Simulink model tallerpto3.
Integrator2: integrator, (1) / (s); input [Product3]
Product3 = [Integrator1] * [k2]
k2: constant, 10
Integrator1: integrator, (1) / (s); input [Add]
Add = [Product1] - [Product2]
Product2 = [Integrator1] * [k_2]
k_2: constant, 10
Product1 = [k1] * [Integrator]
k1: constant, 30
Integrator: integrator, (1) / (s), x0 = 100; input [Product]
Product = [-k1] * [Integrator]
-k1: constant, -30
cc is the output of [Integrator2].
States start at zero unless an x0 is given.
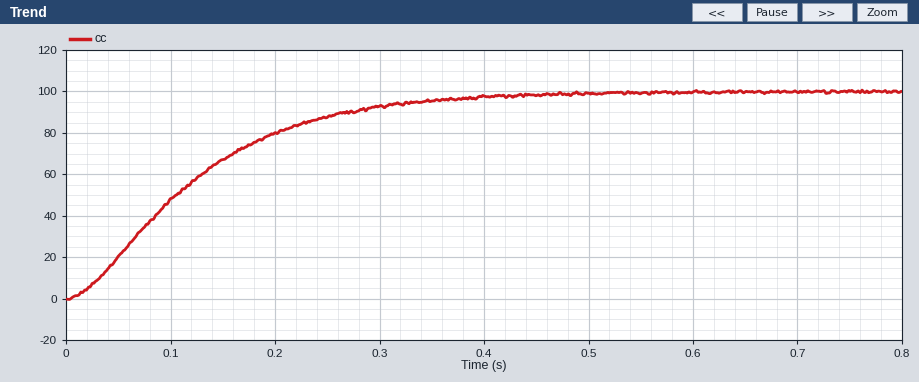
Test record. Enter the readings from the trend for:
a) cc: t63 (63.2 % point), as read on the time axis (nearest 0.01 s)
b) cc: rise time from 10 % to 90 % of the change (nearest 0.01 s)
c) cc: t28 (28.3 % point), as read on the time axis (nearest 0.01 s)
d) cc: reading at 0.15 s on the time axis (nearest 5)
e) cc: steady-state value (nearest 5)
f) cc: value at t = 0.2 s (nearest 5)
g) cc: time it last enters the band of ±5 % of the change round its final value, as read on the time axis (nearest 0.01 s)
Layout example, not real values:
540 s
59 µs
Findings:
0.14 s
0.24 s
0.06 s
65
100
80
0.34 s
